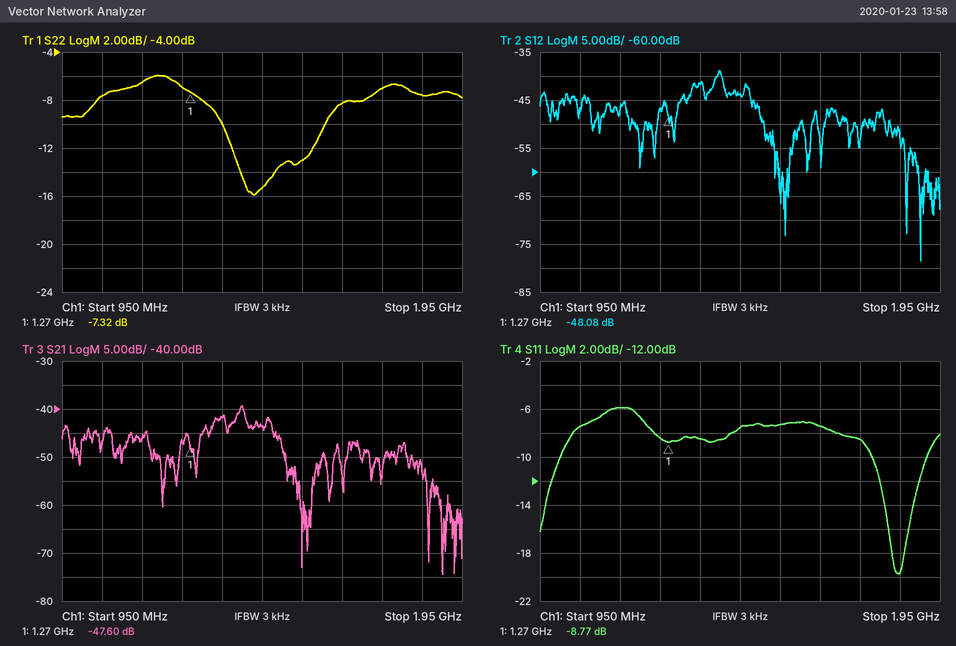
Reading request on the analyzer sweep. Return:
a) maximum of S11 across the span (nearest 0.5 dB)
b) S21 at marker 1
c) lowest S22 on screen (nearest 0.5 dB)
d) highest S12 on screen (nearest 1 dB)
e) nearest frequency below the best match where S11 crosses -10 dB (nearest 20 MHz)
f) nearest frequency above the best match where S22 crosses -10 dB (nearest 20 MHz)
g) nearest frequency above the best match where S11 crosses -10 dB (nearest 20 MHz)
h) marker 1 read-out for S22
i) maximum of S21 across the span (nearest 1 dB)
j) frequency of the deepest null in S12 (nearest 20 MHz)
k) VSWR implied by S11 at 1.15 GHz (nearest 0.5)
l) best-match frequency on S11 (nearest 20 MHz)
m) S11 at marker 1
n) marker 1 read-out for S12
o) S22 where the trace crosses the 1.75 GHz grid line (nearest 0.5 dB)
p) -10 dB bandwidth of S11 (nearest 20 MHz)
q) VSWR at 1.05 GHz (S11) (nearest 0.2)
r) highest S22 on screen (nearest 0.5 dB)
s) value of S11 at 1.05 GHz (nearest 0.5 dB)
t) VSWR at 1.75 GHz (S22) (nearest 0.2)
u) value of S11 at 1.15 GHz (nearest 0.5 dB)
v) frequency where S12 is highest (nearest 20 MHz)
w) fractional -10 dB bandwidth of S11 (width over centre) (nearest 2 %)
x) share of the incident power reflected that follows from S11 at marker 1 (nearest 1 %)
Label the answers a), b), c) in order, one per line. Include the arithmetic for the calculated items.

a) -6.0 dB
b) -47.60 dB
c) -16.0 dB
d) -39 dB
e) 1.78 GHz
f) 1.60 GHz
g) 1.92 GHz
h) -7.32 dB
i) -39 dB
j) 1.90 GHz
k) |Γ| = 10^(-6/20) = 0.5012; VSWR = (1 + 0.5012)/(1 − 0.5012) ≈ 3.0
l) 1.84 GHz
m) -8.77 dB
n) -48.08 dB
o) -7.0 dB
p) 1.92 GHz − 1.78 GHz = 140 MHz
q) |Γ| = 10^(-7.5/20) = 0.4217; VSWR = (1 + 0.4217)/(1 − 0.4217) ≈ 2.46, so 2.4 to the nearest 0.2
r) -6.0 dB
s) -7.5 dB
t) |Γ| = 10^(-7/20) = 0.4467; VSWR = (1 + 0.4467)/(1 − 0.4467) ≈ 2.6
u) -6.0 dB
v) 1.40 GHz
w) 140 MHz / 1.85 GHz ≈ 8 %
x) 10^(-8.77/10) ≈ 13 %
